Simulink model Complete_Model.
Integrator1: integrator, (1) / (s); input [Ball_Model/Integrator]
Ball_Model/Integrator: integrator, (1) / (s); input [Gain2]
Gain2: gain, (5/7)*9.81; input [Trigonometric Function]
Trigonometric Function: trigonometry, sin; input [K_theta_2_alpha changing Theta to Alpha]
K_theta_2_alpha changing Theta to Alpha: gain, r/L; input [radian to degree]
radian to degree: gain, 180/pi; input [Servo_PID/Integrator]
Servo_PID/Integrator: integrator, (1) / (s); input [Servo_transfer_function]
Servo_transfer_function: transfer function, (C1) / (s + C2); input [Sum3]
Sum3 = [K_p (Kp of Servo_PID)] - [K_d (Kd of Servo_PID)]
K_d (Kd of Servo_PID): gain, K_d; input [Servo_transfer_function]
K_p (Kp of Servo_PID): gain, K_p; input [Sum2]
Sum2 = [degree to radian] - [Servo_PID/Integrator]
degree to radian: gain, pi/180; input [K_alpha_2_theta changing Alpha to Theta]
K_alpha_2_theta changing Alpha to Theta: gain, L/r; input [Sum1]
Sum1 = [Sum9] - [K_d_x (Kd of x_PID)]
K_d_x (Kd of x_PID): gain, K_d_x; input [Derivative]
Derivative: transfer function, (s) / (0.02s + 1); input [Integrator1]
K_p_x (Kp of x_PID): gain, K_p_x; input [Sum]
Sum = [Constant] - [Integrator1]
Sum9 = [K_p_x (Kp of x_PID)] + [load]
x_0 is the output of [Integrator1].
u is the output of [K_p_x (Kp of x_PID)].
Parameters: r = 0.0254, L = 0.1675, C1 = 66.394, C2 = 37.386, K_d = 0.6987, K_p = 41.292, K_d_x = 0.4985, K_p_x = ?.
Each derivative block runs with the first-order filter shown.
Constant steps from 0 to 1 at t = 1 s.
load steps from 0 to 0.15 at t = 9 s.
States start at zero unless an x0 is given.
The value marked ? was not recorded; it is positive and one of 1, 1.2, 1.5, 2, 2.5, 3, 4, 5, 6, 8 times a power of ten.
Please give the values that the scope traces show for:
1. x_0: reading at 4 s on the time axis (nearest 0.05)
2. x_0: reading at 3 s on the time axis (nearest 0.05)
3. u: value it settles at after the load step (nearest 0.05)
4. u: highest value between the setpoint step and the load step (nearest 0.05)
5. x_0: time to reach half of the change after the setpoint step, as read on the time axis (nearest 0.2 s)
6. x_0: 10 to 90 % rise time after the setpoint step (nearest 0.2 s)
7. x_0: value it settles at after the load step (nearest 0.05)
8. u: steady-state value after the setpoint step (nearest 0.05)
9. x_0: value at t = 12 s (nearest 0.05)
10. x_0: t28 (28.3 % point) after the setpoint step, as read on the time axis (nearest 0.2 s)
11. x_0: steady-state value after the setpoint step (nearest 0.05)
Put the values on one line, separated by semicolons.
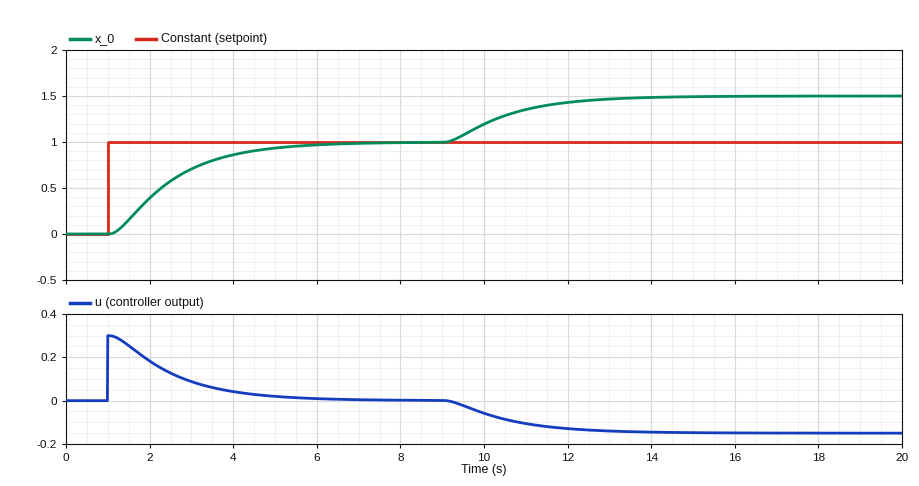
0.85; 0.70; -0.15; 0.30; 2.2 s; 3.0 s; 1.50; 0.00; 1.45; 1.8 s; 1.00
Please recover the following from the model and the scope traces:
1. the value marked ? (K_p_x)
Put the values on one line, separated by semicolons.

0.3
